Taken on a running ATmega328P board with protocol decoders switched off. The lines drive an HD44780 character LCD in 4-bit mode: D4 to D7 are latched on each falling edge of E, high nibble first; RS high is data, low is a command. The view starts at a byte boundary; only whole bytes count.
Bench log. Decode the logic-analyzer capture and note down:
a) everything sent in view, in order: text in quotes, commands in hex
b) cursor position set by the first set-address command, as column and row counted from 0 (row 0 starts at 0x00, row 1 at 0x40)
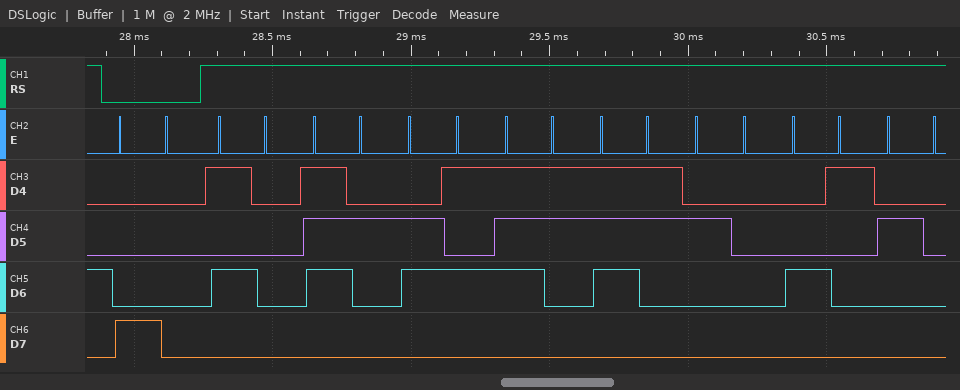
0x80 "Press A "
column 0, row 0
